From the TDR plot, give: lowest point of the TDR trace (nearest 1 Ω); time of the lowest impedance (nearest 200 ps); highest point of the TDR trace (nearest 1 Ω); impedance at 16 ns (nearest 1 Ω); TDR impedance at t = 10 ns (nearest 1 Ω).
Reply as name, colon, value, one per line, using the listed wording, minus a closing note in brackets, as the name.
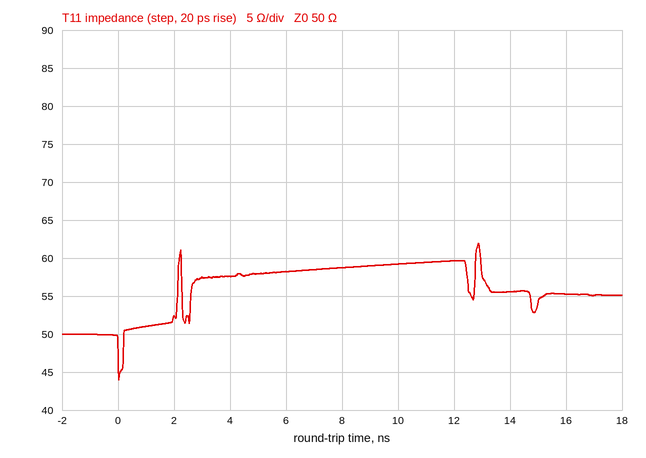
lowest point of the TDR trace: 44 Ω
time of the lowest impedance: 0.0 ns
highest point of the TDR trace: 62 Ω
impedance at 16 ns: 55 Ω
TDR impedance at t = 10 ns: 59 Ω
